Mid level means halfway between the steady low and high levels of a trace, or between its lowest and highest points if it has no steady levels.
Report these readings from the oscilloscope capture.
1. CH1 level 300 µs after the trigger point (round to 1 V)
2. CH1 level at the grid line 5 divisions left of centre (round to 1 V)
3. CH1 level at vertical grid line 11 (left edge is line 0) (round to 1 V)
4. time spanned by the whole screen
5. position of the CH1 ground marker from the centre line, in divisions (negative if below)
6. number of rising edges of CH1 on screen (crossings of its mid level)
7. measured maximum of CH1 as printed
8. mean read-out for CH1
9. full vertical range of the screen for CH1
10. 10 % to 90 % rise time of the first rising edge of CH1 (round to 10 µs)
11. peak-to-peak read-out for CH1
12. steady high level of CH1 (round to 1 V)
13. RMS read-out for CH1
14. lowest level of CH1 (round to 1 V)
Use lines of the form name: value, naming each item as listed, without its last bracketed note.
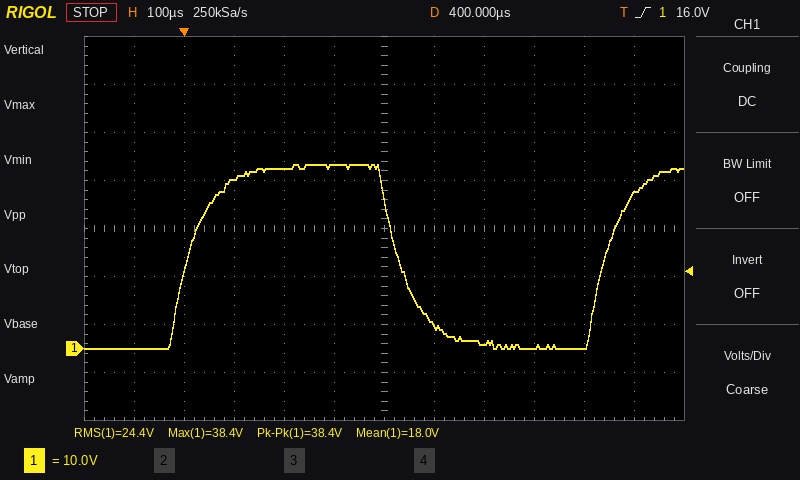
CH1 level 300 µs after the trigger point: 38 V
CH1 level at the grid line 5 divisions left of centre: 0 V
CH1 level at vertical grid line 11 (left edge is line 0): 32 V
time spanned by the whole screen: 1.2 ms
position of the CH1 ground marker from the centre line, in divisions: -2.5 div
number of rising edges of CH1 on screen: 2
measured maximum of CH1 as printed: 38.4 V
mean read-out for CH1: 18.0 V
full vertical range of the screen for CH1: 80 V
10 % to 90 % rise time of the first rising edge of CH1: 110 µs
peak-to-peak read-out for CH1: 38.4 V
steady high level of CH1: 38 V
RMS read-out for CH1: 24.4 V
lowest level of CH1: 0 V
